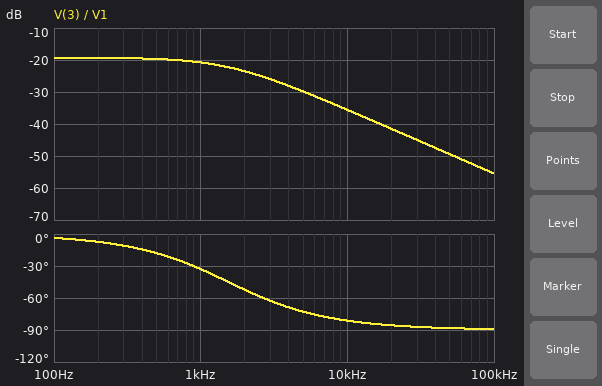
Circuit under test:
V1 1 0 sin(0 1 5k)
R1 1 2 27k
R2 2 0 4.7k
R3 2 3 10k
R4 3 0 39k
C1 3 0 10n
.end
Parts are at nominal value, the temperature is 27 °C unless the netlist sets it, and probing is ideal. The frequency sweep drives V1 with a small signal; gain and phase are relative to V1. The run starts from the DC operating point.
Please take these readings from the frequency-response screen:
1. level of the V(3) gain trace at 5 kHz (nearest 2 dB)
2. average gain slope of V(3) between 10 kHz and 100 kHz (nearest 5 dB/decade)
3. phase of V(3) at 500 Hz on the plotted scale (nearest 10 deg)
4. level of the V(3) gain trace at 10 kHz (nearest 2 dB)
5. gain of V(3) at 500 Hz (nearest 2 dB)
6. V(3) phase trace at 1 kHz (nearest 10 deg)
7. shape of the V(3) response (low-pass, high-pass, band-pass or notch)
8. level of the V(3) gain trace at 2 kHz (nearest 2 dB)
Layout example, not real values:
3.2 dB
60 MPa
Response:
-30 dB
-20 dB/decade
-20 deg
-36 dB
-20 dB
-30 deg
low-pass
-24 dB
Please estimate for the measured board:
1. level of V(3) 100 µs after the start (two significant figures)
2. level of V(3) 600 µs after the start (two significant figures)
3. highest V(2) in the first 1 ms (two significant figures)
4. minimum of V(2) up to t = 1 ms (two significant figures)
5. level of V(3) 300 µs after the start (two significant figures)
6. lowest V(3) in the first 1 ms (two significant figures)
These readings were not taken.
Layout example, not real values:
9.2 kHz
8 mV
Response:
42 mV
-31 mV
110 mV
-110 mV
32 mV
-32 mV
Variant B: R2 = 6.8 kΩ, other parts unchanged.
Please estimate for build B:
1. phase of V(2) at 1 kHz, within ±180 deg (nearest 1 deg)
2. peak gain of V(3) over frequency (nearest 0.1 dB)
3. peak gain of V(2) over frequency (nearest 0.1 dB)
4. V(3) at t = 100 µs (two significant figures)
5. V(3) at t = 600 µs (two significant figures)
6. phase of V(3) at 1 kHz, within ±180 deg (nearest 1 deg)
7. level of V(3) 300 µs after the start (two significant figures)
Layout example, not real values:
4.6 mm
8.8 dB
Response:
-8 deg
-16.8 dB
-14.8 dB
54 mV
-38 mV
-35 deg
41 mV
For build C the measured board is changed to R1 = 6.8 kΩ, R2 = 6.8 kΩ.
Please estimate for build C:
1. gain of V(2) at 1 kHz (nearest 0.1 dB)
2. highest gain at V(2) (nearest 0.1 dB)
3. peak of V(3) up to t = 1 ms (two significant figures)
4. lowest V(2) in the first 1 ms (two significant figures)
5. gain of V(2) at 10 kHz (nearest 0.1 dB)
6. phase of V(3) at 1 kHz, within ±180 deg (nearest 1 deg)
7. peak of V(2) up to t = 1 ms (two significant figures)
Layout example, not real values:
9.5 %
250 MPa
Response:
-7.1 dB
-6.6 dB
160 mV
-380 mV
-8.5 dB
-32 deg
400 mV
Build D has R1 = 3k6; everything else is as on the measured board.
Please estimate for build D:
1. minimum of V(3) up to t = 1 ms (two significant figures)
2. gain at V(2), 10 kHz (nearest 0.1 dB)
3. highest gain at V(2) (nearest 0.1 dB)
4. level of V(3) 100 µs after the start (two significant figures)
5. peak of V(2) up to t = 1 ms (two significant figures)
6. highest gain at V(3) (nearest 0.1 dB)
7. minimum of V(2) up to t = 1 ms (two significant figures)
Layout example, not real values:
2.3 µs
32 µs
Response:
-140 mV
-6.5 dB
-5.3 dB
180 mV
490 mV
-7.3 dB
-480 mV
